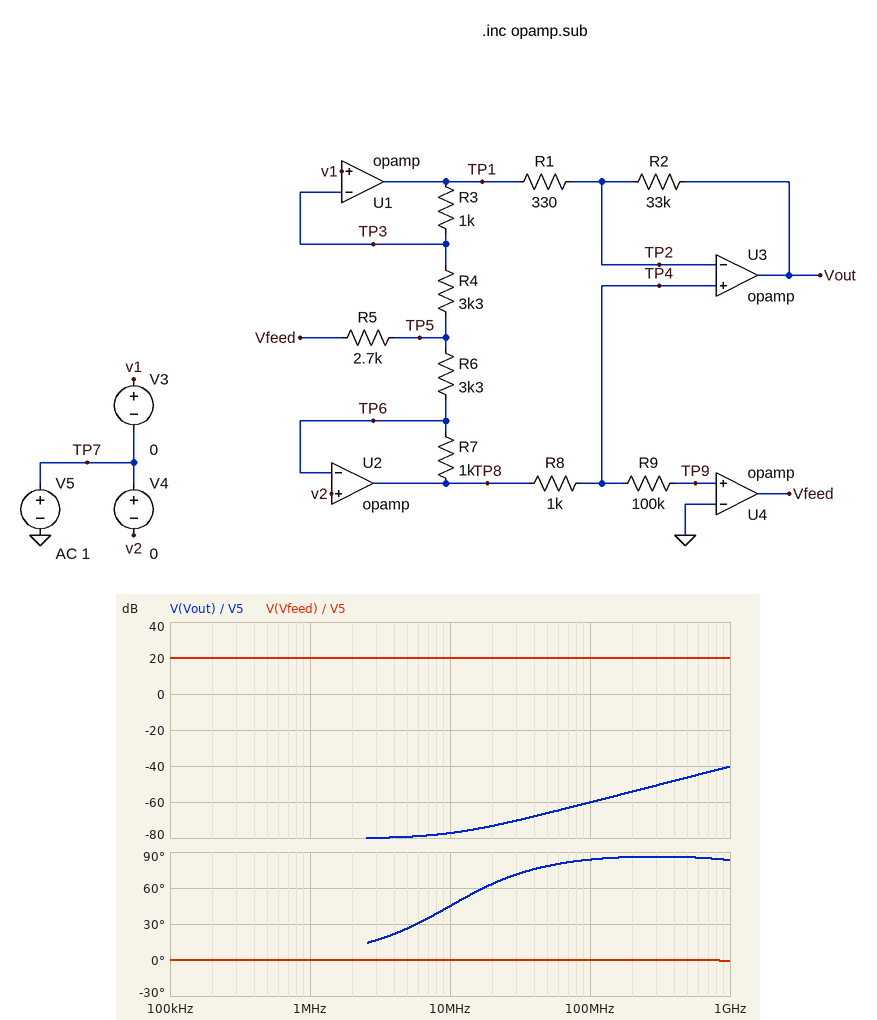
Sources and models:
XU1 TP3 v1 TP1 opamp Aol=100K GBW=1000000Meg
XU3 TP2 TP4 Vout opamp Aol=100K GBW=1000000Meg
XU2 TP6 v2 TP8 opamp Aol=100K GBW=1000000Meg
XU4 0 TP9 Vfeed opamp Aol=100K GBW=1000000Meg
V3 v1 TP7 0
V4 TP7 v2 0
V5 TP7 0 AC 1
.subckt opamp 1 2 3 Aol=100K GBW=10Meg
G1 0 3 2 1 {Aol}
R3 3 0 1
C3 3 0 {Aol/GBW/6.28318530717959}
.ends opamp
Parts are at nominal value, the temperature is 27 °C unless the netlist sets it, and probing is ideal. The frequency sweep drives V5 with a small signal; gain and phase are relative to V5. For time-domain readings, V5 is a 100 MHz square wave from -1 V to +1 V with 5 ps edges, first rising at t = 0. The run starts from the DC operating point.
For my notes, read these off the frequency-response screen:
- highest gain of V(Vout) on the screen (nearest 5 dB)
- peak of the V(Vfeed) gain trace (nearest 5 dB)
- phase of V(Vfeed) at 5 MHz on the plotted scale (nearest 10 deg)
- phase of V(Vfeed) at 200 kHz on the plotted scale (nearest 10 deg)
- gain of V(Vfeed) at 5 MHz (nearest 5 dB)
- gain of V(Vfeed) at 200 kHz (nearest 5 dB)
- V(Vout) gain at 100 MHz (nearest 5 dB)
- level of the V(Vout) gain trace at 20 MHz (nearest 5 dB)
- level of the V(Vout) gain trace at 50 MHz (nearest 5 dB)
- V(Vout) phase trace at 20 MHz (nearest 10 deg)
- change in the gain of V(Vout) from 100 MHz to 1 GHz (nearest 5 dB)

-40 dB
20 dB
0 deg
0 deg
20 dB
20 dB
-60 dB
-75 dB
-65 dB
60 deg
20 dB
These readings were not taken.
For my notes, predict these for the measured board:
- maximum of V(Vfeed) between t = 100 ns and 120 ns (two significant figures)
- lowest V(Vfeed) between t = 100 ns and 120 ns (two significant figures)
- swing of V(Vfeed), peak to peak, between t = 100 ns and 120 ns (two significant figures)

9.7 V
-9.7 V
19 V
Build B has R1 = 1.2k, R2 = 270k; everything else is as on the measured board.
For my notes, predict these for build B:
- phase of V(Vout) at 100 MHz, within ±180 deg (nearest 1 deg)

83 deg
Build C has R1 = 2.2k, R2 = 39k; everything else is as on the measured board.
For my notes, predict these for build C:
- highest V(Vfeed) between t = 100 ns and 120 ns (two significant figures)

9.7 V
